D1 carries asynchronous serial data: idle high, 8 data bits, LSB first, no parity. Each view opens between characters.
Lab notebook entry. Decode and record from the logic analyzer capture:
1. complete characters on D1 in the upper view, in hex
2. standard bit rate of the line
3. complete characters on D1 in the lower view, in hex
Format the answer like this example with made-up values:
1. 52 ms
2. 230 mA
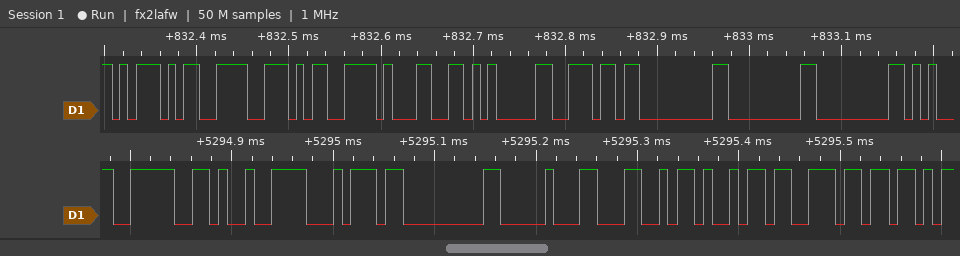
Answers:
1. 5D, 9E, CD, 31, 05, 6E, 00, 00, 00
2. 115200 baud
3. 3E, C9, 74, 00, 10, 4C, 69, 6E
